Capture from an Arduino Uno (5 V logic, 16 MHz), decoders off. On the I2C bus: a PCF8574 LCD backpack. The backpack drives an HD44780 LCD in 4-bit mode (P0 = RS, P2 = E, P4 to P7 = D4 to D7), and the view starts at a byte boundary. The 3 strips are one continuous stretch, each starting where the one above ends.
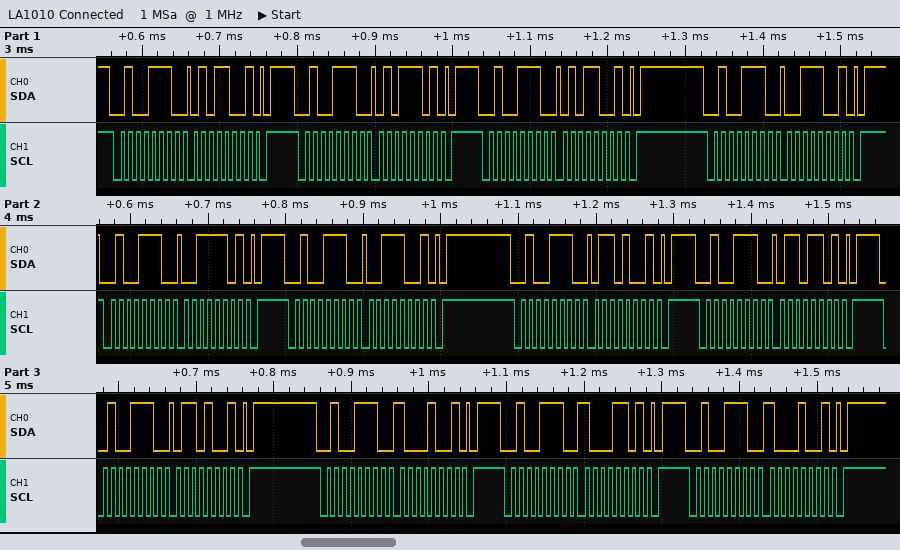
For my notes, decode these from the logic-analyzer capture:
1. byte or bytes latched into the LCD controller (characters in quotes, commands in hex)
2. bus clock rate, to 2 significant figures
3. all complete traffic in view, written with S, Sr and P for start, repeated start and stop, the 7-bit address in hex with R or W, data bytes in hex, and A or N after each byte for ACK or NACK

'S' 'h'
100 kHz
S 27W A 59 A P S 27W A 5D A P S 27W A 59 A P S 27W A 39 A P S 27W A 3D A P S 27W A 39 A P S 27W A 69 A P S 27W A 6D A P S 27W A 69 A P S 27W A 89 A P S 27W A 8D A P S 27W A 89 A P
